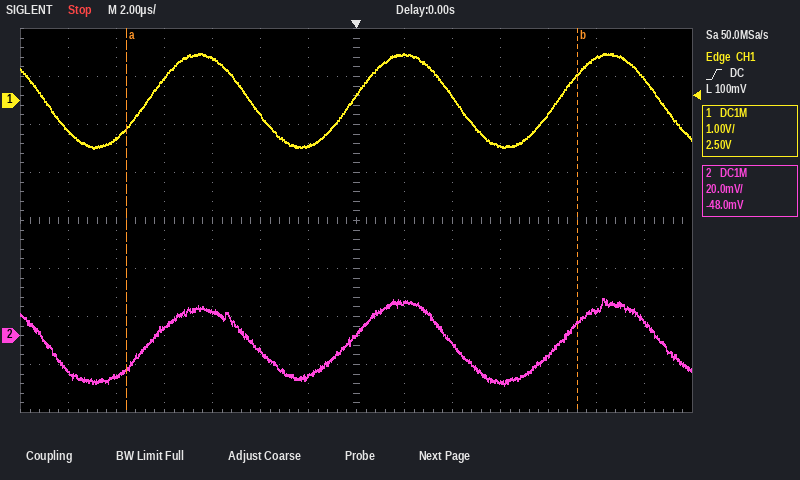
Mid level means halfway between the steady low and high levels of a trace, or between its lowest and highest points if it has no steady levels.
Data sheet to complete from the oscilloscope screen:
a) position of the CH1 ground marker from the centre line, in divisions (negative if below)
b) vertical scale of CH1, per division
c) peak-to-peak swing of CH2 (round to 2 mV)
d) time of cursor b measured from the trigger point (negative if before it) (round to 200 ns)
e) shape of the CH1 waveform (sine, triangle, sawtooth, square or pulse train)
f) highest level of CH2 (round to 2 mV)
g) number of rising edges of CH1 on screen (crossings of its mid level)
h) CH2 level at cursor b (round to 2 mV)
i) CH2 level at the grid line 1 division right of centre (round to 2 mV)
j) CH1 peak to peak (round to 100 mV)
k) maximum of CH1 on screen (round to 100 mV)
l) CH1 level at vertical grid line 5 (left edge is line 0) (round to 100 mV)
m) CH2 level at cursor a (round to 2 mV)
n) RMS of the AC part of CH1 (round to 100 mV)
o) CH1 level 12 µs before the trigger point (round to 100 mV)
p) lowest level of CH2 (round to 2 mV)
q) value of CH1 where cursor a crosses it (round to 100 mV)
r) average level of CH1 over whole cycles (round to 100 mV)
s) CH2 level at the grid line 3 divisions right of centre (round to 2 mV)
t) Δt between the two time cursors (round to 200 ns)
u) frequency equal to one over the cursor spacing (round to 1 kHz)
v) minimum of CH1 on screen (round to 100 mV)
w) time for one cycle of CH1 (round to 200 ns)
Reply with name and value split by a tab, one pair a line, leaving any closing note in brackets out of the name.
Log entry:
position of the CH1 ground marker from the centre line, in divisions	+2.5 div
vertical scale of CH1, per division	1 V
peak-to-peak swing of CH2	36 mV
time of cursor b measured from the trigger point (negative if before it)	+9.2 µs
shape of the CH1 waveform	sine
highest level of CH2	16 mV
number of rising edges of CH1 on screen	3
CH2 level at cursor b	6 mV
CH2 level at the grid line 1 division right of centre	14 mV
CH1 peak to peak	2.0 V
maximum of CH1 on screen	1.0 V
CH1 level at vertical grid line 5 (left edge is line 0)	-300 mV
CH2 level at cursor a	-14 mV
RMS of the AC part of CH1	700 mV
CH1 level 12 µs before the trigger point	-600 mV
lowest level of CH2	-20 mV
value of CH1 where cursor a crosses it	-600 mV
average level of CH1 over whole cycles	0.0 V
CH2 level at the grid line 3 divisions right of centre	-20 mV
Δt between the two time cursors	18.8 µs
frequency equal to one over the cursor spacing	53 kHz
minimum of CH1 on screen	-1.0 V
time for one cycle of CH1	8.6 µs
